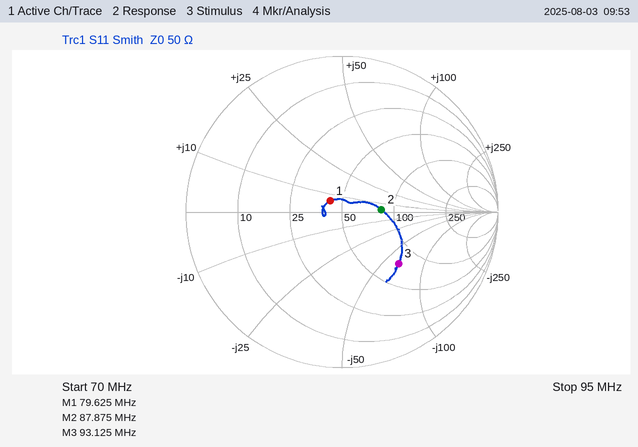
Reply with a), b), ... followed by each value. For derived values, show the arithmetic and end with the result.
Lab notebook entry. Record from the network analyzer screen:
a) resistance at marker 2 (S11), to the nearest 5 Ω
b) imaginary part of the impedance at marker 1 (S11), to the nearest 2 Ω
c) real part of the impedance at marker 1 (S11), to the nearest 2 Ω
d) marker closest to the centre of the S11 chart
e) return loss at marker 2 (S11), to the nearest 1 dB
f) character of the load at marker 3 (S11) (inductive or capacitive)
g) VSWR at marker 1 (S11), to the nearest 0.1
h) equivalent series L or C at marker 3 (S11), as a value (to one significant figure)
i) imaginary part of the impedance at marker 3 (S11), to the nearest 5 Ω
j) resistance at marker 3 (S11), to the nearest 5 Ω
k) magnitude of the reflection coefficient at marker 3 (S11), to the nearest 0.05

a) 85 Ω
b) +6 Ω
c) 42 Ω
d) marker 1
e) 12 dB
f) capacitive
g) 1.2
h) C = 1/(2π × 93.125 MHz × 65 Ω) ≈ 26.3 pF, so 30 pF to one significant figure
i) -65 Ω
j) 75 Ω
k) 0.50
